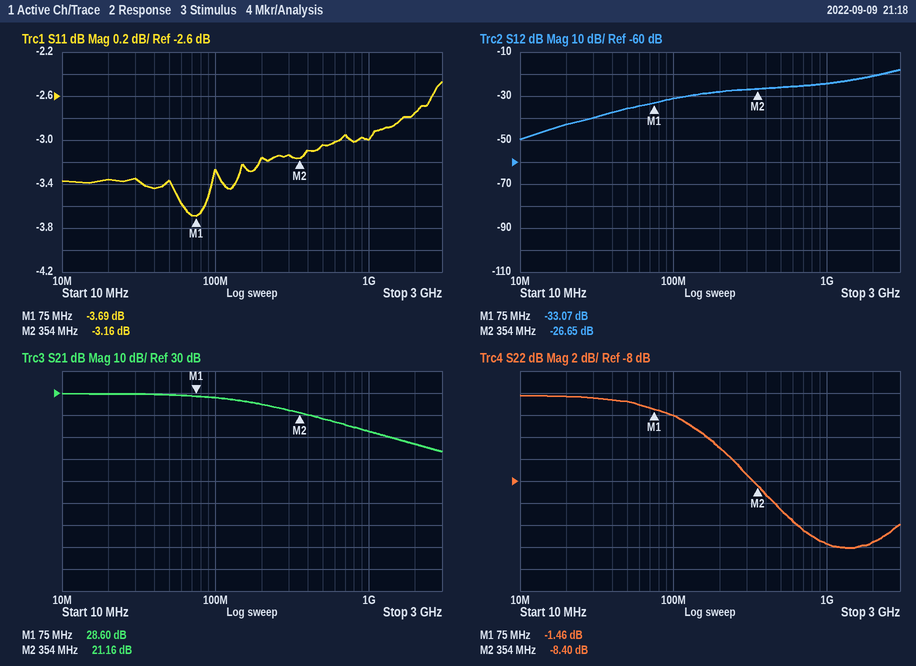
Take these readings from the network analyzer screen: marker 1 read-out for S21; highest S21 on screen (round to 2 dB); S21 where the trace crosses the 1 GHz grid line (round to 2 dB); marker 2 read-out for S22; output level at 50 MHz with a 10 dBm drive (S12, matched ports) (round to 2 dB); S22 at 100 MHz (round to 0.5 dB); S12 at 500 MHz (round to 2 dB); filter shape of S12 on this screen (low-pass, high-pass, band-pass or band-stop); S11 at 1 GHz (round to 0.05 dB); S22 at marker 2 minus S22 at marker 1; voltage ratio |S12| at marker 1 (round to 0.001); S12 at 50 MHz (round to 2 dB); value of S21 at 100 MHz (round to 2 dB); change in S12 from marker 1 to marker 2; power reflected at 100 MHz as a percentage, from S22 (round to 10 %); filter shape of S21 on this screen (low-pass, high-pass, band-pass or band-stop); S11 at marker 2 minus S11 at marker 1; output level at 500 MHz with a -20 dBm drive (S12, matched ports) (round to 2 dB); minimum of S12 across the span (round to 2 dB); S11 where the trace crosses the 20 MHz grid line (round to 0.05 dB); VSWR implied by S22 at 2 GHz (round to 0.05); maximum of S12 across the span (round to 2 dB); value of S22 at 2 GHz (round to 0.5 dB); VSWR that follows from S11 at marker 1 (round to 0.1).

28.60 dB
30 dB
12 dB
-8.40 dB
-26 dBm
-2.0 dB
-26 dB
high-pass
-3.00 dB
-6.94 dB
0.022
-36 dB
28 dB
6.42 dB
60 %
low-pass
0.53 dB
-46 dBm
-50 dB
-3.35 dB
1.55
-18 dB
-13.5 dB
4.8
